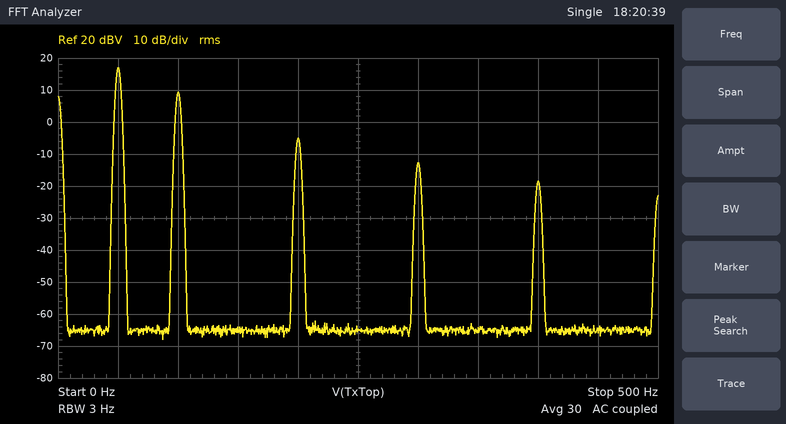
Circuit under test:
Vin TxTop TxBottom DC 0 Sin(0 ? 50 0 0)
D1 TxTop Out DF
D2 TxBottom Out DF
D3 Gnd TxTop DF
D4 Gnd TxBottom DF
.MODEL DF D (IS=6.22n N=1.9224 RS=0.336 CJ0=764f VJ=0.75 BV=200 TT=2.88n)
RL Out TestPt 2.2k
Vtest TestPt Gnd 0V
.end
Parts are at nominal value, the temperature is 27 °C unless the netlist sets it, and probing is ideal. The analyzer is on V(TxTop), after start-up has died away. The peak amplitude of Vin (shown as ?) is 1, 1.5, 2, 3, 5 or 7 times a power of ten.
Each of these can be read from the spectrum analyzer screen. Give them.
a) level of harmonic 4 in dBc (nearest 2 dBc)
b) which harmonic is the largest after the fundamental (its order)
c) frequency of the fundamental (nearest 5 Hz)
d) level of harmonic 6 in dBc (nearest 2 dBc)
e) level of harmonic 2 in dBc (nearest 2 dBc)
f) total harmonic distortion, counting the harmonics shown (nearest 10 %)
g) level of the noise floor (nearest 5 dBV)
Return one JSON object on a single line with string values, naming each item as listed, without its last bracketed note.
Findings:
{"level of harmonic 4 in dBc": "-22 dBc", "which harmonic is the largest after the fundamental": "2", "frequency of the fundamental": "50 Hz", "level of harmonic 6 in dBc": "-30 dBc", "level of harmonic 2 in dBc": "-8 dBc", "total harmonic distortion, counting the harmonics shown": "40 %", "level of the noise floor": "-65 dBV"}
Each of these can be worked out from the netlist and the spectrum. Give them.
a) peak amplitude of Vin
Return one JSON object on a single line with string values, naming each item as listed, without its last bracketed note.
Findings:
{"peak amplitude of Vin": "20 V"}
